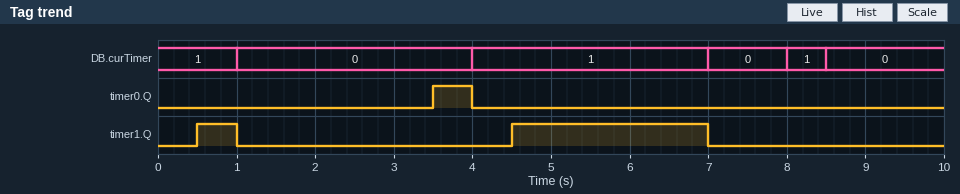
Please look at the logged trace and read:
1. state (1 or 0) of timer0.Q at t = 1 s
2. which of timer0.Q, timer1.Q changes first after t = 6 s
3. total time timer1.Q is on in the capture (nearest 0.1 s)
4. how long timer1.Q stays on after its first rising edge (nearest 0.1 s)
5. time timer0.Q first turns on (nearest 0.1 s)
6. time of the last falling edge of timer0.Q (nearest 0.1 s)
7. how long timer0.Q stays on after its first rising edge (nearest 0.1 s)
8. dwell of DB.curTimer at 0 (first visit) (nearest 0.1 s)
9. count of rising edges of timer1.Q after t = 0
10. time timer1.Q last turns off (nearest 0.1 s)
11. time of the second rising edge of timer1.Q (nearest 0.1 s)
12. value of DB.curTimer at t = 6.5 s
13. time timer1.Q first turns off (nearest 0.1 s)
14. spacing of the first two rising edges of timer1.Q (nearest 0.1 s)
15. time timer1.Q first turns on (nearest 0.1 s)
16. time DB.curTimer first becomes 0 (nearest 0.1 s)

0
timer1.Q
3.0 s
0.5 s
3.5 s
4.0 s
0.5 s
3.0 s
2
7.0 s
4.5 s
1
1.0 s
4.0 s
0.5 s
1.0 s
